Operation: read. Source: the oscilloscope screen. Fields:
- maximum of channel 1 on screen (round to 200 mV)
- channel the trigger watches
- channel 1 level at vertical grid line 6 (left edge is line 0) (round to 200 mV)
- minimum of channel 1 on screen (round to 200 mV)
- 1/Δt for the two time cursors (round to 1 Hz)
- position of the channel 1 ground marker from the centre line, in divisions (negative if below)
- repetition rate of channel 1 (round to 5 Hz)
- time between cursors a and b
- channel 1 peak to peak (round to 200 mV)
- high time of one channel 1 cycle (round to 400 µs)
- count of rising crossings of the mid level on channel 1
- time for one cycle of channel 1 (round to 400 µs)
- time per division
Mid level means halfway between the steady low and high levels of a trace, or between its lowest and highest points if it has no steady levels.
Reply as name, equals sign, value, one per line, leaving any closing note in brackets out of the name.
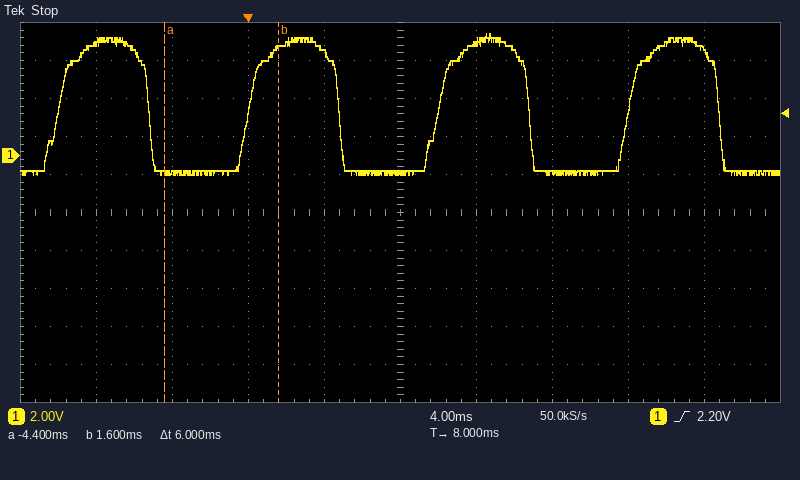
maximum of channel 1 on screen = 6.4 V
channel the trigger watches = channel 1
channel 1 level at vertical grid line 6 (left edge is line 0) = 6.0 V
minimum of channel 1 on screen = -1.0 V
1/Δt for the two time cursors = 167 Hz
position of the channel 1 ground marker from the centre line, in divisions = +1.5 div
repetition rate of channel 1 = 100 Hz
time between cursors a and b = 6 ms
channel 1 peak to peak = 7.4 V
high time of one channel 1 cycle = 4.8 ms
count of rising crossings of the mid level on channel 1 = 4
time for one cycle of channel 1 = 10.0 ms
time per division = 4 ms
